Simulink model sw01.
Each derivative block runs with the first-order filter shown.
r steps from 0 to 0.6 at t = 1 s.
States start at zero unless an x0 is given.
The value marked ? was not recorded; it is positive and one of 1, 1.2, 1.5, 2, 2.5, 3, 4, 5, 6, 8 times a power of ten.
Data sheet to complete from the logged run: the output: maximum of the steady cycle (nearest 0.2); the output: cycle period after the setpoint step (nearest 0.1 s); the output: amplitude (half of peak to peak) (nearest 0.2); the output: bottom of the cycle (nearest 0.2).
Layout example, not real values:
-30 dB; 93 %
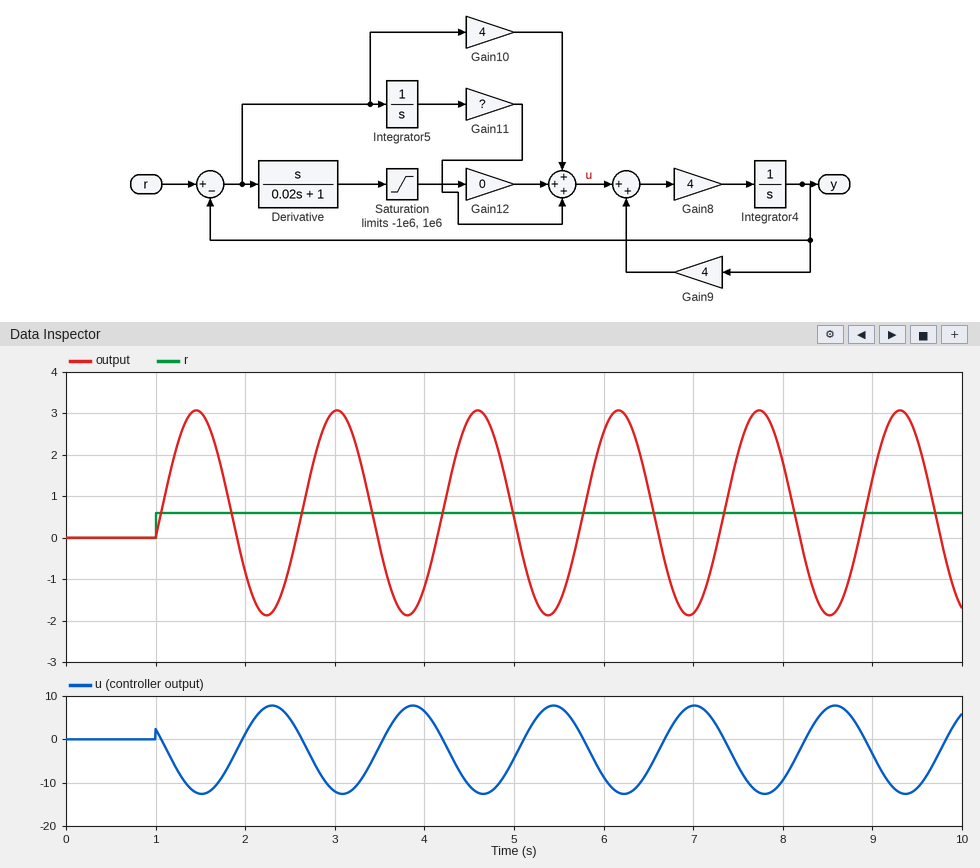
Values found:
3.0; 1.6 s; 2.4; -1.8
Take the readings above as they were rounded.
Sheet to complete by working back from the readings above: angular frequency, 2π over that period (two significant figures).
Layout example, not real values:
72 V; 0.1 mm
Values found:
3.9 rad/s
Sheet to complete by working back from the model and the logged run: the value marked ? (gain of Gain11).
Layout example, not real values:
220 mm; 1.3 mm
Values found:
4
